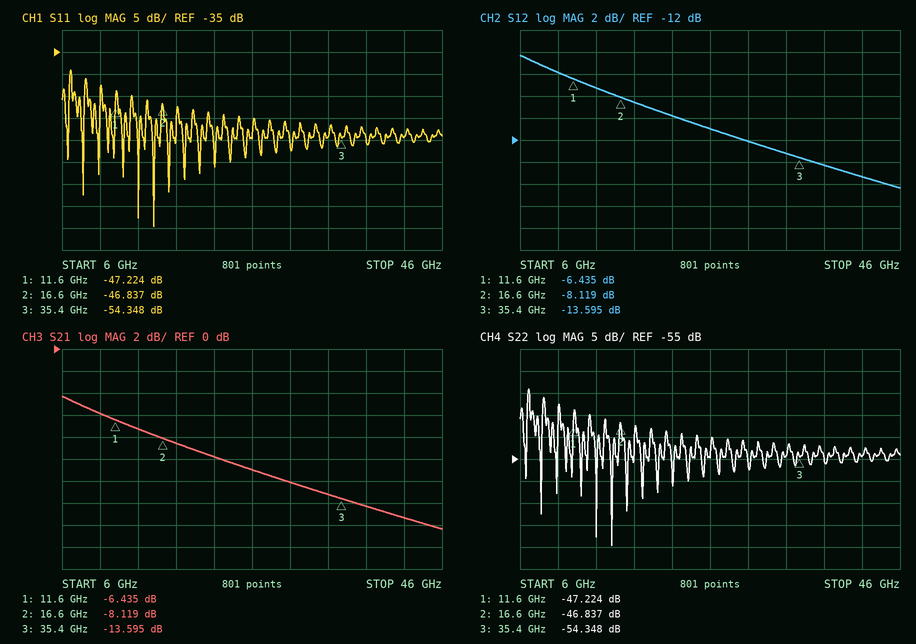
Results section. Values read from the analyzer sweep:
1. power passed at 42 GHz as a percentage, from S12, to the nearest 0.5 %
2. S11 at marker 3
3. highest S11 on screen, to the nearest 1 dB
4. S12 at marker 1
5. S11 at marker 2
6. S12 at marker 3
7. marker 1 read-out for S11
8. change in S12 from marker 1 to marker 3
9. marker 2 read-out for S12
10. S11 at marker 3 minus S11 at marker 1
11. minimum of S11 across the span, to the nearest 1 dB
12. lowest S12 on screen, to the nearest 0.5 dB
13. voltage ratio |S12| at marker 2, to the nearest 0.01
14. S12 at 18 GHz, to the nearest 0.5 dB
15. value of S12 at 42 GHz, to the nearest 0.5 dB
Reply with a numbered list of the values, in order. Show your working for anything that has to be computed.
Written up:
1. 10^(-15.5/10) ≈ 2.82 %, so 3.0 % to the nearest 0.5 %
2. -54.348 dB
3. -39 dB
4. -6.435 dB
5. -46.837 dB
6. -13.595 dB
7. -47.224 dB
8. -13.595 − (-6.435) = -7.160 dB
9. -8.119 dB
10. -54.348 − (-47.224) = -7.124 dB
11. -75 dB
12. -16.5 dB
13. 10^(-8.119/20) ≈ 0.39
14. -8.5 dB
15. -15.5 dB
